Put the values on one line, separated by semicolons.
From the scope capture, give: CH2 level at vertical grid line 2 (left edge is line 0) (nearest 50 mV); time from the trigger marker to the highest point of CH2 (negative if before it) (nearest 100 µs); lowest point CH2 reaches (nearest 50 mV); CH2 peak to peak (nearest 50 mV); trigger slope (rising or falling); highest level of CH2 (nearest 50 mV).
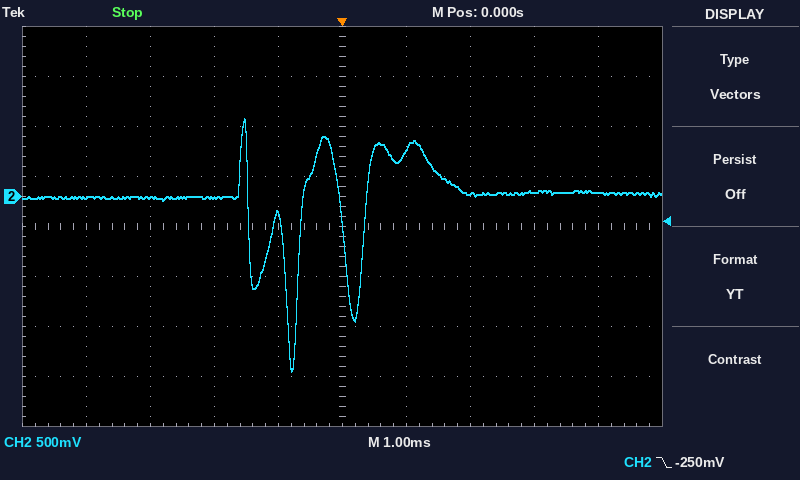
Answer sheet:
0 mV; -1.5 ms; -1.75 V; 2.55 V; falling; 800 mV
